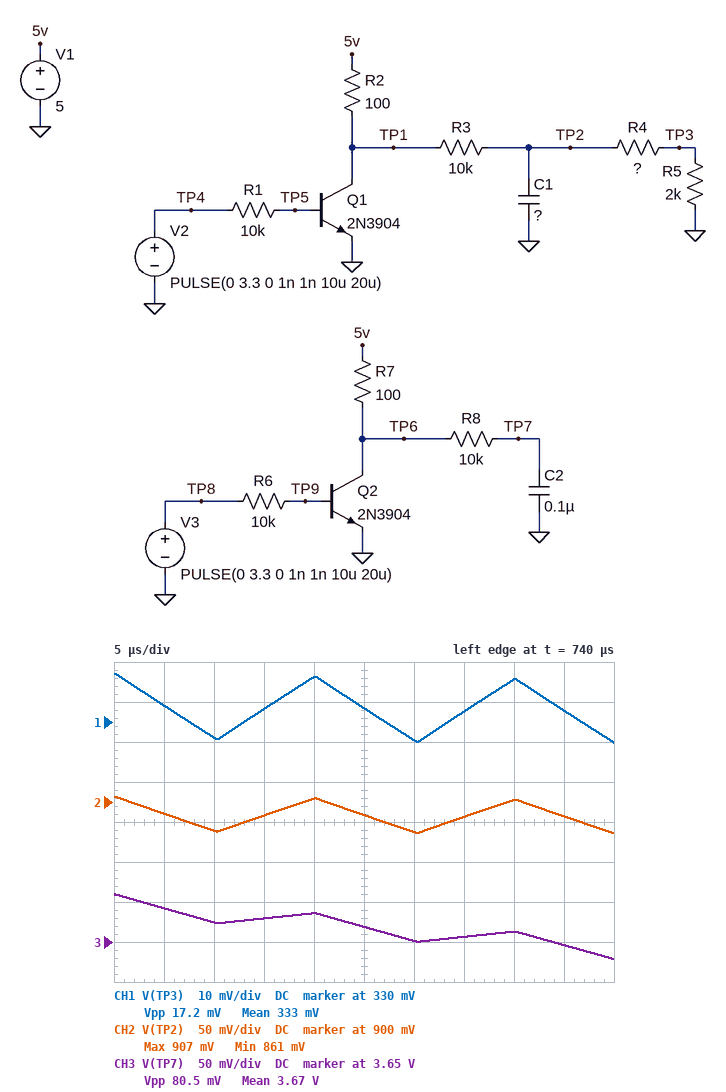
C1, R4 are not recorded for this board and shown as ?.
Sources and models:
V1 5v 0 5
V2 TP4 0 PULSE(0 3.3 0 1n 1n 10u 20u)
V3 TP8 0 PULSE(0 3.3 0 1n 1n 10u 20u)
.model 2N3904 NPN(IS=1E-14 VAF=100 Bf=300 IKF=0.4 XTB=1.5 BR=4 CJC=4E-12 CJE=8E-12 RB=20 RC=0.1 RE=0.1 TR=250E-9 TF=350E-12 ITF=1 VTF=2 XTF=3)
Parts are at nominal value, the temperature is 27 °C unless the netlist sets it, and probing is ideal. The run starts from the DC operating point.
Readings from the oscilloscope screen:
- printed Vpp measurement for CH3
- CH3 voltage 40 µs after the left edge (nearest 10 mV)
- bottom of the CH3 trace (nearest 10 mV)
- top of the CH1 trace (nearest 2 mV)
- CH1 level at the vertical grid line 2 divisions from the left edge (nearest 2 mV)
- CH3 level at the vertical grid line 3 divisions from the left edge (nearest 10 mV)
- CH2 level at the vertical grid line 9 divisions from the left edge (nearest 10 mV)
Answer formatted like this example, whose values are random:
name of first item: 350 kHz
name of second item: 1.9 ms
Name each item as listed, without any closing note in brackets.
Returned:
printed Vpp measurement for CH3: 80.5 mV
CH3 voltage 40 µs after the left edge: 3.66 V
bottom of the CH3 trace: 3.63 V
top of the CH1 trace: 342 mV
CH1 level at the vertical grid line 2 divisions from the left edge: 326 mV
CH3 level at the vertical grid line 3 divisions from the left edge: 3.68 V
CH2 level at the vertical grid line 9 divisions from the left edge: 880 mV
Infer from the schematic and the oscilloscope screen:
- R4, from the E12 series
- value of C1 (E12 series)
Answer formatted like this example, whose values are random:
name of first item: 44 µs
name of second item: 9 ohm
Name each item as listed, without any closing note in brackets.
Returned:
R4, from the E12 series: 3.3 kΩ
value of C1: 56 nF
